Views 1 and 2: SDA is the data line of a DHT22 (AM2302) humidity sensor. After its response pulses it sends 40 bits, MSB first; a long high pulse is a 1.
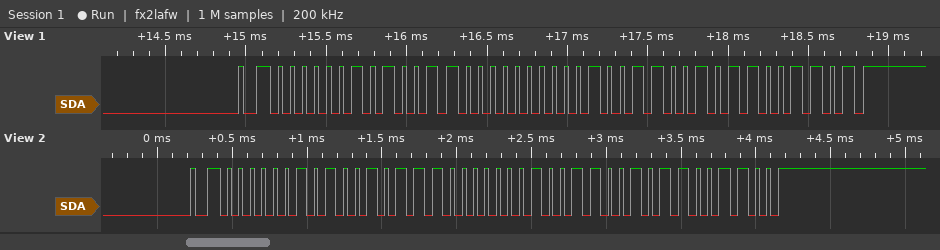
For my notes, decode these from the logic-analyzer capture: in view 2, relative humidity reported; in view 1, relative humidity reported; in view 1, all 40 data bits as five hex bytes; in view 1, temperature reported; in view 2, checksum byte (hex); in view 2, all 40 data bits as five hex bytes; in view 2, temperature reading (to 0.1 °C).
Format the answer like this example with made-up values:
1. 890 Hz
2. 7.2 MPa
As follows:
1. 66.3 %
2. 66.4 %
3. 02 98 01 32 CD
4. 30.6 °C
5. 0xCC
6. 02 97 01 32 CC
7. 30.6 °C
